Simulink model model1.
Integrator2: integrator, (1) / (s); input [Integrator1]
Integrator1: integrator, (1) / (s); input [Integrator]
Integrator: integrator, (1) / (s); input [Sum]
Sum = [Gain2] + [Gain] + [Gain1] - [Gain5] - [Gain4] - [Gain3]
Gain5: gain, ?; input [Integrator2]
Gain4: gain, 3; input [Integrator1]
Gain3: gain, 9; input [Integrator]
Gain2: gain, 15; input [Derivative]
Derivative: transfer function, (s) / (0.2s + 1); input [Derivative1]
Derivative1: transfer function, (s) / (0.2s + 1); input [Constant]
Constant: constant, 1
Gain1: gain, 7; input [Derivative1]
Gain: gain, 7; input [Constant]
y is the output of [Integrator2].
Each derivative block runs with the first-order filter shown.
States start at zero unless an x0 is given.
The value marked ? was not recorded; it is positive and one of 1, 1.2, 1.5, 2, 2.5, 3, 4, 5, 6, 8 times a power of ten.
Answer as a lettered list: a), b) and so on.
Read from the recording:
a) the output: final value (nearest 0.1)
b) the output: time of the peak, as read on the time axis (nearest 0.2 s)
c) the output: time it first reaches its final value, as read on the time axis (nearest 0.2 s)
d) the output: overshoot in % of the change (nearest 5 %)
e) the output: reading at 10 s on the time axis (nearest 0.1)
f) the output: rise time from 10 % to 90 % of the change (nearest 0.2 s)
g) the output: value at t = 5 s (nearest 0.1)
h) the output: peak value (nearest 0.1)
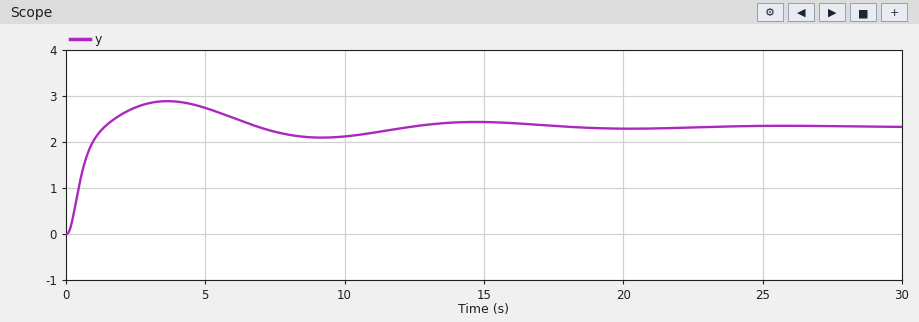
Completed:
a) 2.3
b) 3.6 s
c) 1.4 s
d) 25 %
e) 2.1
f) 0.8 s
g) 2.7
h) 2.9
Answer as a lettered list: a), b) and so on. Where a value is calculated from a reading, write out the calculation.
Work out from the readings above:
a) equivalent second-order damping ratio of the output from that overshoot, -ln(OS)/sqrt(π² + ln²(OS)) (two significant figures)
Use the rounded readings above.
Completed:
a) ln(0.25) = -1.386; 1.386 / sqrt(9.870 + 1.922) = 0.40
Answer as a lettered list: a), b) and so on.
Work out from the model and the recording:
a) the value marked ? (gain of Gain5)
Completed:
a) 3
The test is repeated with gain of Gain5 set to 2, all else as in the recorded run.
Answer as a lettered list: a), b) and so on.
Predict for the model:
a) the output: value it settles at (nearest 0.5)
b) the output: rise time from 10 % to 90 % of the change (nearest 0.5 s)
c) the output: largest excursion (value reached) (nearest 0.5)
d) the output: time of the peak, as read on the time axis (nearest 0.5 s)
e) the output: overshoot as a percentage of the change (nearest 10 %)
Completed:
a) 3.5
b) 2.5 s
c) 4.0
d) 6.0 s
e) 20 %
